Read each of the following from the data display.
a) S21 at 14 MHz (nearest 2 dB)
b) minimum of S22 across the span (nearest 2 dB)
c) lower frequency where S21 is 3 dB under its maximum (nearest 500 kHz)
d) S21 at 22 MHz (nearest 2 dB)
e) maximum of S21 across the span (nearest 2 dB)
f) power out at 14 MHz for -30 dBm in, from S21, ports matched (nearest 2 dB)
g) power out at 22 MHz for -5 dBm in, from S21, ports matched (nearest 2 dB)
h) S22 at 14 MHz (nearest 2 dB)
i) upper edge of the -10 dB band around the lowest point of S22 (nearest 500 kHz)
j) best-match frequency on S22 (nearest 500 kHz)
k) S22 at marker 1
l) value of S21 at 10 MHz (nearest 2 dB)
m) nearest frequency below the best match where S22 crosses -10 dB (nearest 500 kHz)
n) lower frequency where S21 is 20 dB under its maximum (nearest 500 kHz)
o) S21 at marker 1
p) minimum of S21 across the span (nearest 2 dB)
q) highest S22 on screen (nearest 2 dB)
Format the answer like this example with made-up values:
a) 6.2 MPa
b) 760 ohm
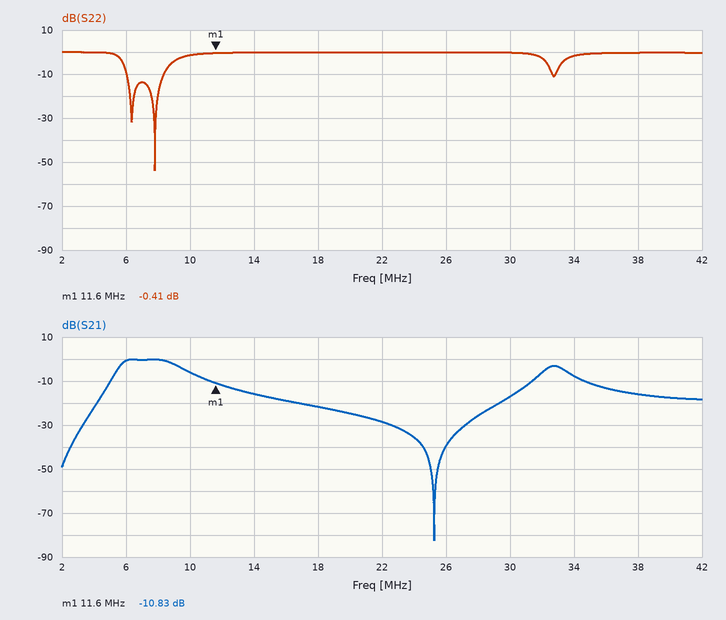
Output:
a) -16 dB
b) -54 dB
c) 5.5 MHz
d) -28 dB
e) 0 dB
f) -46 dBm
g) -34 dBm
h) 0 dB
i) 8.5 MHz
j) 8.0 MHz
k) -0.41 dB
l) -6 dB
m) 6.0 MHz
n) 4.0 MHz
o) -10.83 dB
p) -82 dB
q) 0 dB
